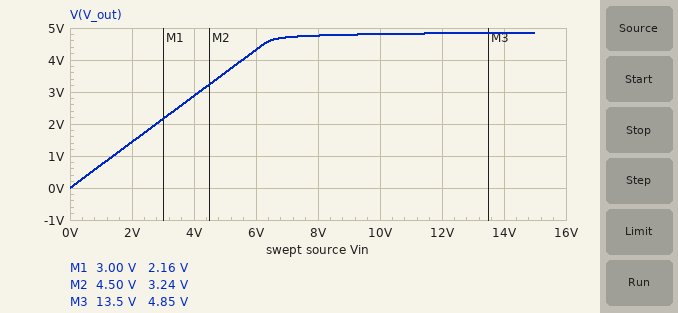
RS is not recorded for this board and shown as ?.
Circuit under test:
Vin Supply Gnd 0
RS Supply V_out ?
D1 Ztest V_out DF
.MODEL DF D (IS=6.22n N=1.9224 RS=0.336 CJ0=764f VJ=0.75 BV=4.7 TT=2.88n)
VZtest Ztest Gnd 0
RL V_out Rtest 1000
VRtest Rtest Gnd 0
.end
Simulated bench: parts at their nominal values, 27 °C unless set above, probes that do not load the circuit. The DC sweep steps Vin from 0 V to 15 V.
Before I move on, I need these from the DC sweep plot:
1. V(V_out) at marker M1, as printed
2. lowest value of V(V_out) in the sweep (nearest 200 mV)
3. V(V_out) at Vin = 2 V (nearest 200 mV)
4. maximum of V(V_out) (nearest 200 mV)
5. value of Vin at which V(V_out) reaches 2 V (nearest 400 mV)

2.16 V
0 V
1.4 V
4.8 V
2.8 V
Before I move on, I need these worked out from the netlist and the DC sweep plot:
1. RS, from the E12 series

390 Ω
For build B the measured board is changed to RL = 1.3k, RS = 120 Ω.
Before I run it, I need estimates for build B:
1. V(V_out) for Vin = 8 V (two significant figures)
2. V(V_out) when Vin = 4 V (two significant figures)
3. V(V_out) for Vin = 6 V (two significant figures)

4.9 V
3.7 V
4.8 V
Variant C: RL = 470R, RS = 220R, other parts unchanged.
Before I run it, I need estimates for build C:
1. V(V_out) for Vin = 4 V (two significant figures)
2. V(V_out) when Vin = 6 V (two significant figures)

2.7 V
4.1 V
